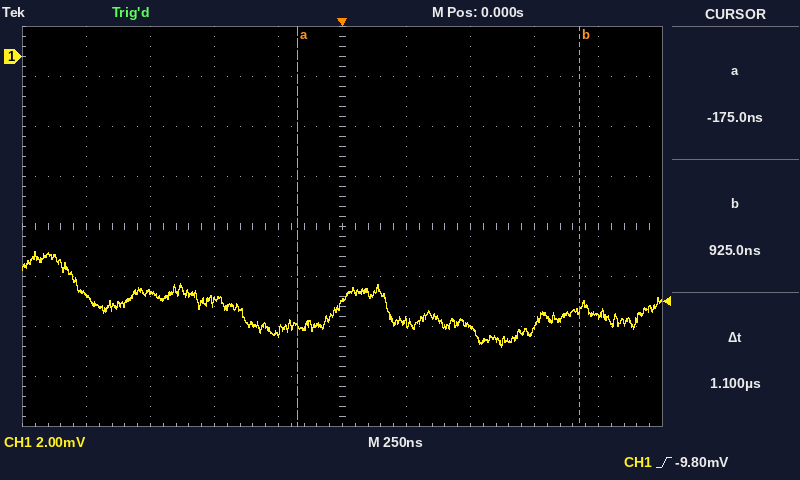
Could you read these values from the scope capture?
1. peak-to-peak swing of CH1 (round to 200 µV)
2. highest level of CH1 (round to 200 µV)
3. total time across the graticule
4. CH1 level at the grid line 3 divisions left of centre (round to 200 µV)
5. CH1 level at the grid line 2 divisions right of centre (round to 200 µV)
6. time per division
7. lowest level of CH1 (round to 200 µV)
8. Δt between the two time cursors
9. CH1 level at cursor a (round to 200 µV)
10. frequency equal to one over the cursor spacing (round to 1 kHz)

3.8 mV
-7.8 mV
2.5 µs
-9.4 mV
-10.8 mV
250 ns
-11.6 mV
1.1 µs
-10.8 mV
909 kHz
